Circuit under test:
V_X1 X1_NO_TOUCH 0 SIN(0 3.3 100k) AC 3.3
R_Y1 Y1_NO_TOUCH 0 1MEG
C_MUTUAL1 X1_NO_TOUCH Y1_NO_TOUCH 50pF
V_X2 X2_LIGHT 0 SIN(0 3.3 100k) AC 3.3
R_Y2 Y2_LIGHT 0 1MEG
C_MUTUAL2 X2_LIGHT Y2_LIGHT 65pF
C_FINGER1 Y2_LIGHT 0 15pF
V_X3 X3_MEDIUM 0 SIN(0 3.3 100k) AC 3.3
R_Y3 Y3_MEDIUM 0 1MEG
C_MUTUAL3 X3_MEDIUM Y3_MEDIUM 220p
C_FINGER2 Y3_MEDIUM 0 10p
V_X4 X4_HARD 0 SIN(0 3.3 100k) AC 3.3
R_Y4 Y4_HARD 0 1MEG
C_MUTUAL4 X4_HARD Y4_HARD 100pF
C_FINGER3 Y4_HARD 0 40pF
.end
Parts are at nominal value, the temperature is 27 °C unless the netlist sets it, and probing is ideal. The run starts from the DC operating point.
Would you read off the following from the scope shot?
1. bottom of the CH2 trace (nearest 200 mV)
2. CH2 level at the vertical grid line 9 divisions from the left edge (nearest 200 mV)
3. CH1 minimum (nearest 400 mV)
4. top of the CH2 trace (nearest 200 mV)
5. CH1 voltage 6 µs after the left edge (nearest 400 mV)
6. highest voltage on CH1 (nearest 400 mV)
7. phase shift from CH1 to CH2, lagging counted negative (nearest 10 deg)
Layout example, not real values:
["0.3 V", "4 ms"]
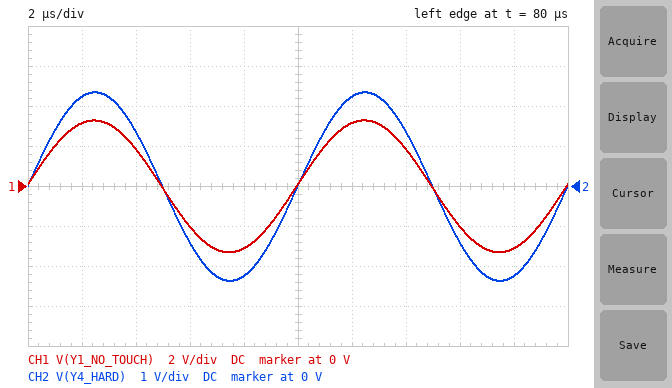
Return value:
["-2.4 V", "-2.2 V", "-3.2 V", "2.4 V", "-2.0 V", "3.2 V", "0 deg"]
